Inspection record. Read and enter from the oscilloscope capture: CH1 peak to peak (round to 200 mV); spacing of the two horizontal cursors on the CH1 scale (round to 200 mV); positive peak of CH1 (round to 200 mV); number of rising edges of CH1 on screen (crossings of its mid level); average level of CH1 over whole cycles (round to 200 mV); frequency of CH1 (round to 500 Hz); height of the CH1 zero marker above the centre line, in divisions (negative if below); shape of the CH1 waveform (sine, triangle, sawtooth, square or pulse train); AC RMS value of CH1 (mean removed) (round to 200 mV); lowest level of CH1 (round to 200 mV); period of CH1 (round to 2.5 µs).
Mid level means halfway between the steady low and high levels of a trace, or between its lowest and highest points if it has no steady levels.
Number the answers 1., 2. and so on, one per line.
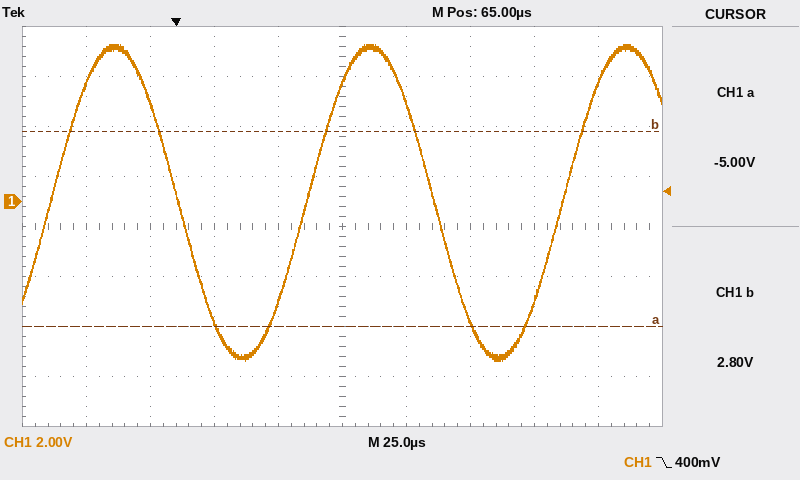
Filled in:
1. 12.6 V
2. 7.8 V
3. 6.2 V
4. 3
5. 0.0 V
6. 10.0 kHz
7. +0.5 div
8. sine
9. 4.4 V
10. -6.4 V
11. 100.0 µs
